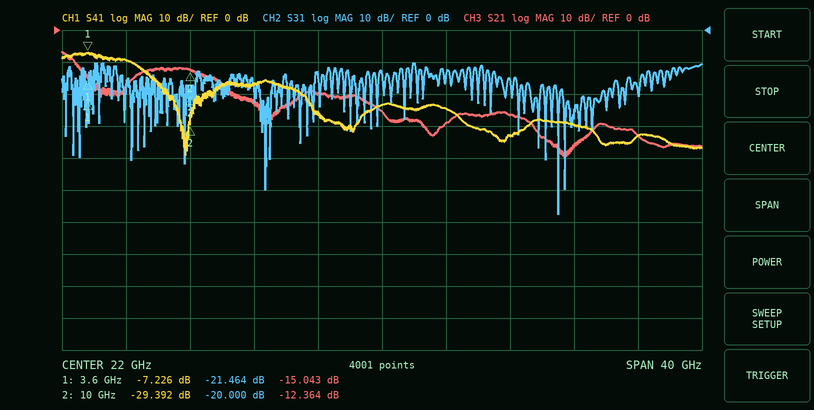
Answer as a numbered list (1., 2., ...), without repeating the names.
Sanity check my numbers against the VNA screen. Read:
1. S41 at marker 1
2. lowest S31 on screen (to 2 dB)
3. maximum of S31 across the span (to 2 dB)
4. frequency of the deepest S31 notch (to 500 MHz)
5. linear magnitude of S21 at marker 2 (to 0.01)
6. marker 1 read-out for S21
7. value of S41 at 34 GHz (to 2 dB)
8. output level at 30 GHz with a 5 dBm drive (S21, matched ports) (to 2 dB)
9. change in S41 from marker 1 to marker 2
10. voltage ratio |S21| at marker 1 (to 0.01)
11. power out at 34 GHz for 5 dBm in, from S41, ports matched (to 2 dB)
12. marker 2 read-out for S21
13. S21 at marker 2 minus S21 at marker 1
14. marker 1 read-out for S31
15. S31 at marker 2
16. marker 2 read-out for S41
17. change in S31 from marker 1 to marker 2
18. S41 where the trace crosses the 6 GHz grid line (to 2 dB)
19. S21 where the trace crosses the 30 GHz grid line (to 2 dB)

1. -7.226 dB
2. -58 dB
3. -10 dB
4. 33.0 GHz
5. 0.24
6. -15.043 dB
7. -30 dB
8. -22 dBm
9. -22.166 dB
10. 0.18
11. -24 dBm
12. -12.364 dB
13. 2.679 dB
14. -21.464 dB
15. -20.000 dB
16. -29.392 dB
17. 1.464 dB
18. -10 dB
19. -26 dB
